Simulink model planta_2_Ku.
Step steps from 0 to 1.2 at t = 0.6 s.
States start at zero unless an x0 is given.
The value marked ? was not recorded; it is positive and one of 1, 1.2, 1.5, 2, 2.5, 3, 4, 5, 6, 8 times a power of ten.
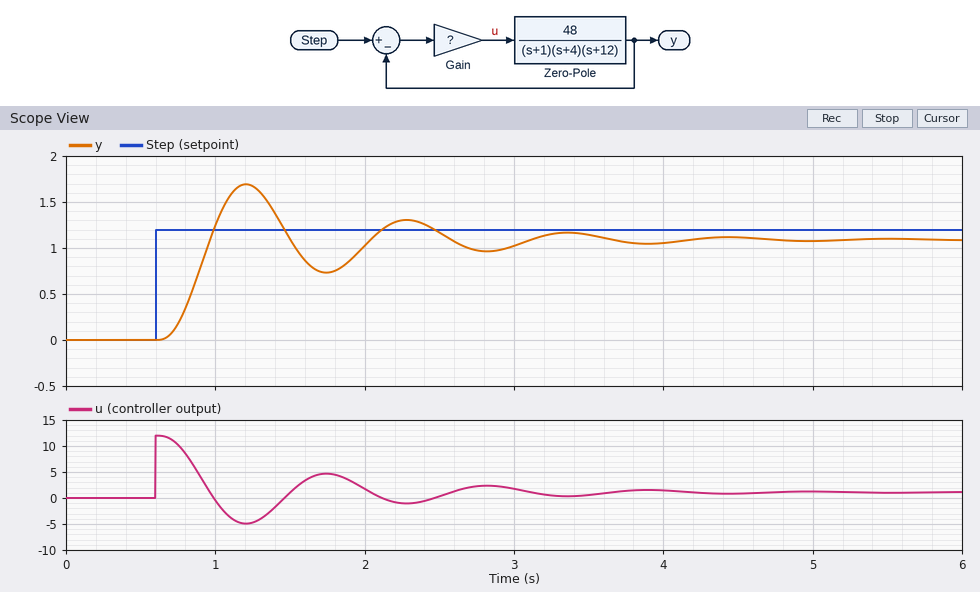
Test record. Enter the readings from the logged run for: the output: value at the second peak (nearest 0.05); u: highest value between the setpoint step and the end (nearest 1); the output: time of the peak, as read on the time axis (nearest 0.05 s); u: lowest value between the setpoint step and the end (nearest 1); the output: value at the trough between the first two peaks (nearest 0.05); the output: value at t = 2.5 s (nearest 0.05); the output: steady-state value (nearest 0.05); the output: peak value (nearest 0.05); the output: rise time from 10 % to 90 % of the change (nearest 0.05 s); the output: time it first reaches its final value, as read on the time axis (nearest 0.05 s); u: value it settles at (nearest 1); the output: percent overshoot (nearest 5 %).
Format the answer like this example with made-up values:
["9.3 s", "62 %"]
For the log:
["1.30", "12", "1.20 s", "-5", "0.75", "1.15", "1.10", "1.70", "0.20 s", "0.95 s", "1", "55 %"]
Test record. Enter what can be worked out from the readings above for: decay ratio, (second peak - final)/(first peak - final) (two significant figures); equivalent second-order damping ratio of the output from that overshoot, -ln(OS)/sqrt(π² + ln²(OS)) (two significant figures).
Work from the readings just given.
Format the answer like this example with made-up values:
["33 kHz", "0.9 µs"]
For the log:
["0.33", "0.19"]
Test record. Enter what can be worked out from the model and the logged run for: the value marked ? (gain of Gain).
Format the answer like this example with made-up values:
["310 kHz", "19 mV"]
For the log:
["10"]
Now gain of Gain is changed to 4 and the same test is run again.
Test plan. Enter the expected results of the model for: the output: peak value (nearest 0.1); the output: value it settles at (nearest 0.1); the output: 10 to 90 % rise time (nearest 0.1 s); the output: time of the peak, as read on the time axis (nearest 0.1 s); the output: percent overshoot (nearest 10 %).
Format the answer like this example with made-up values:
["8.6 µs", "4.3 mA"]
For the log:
["1.2", "1.0", "0.4 s", "1.5 s", "20 %"]
